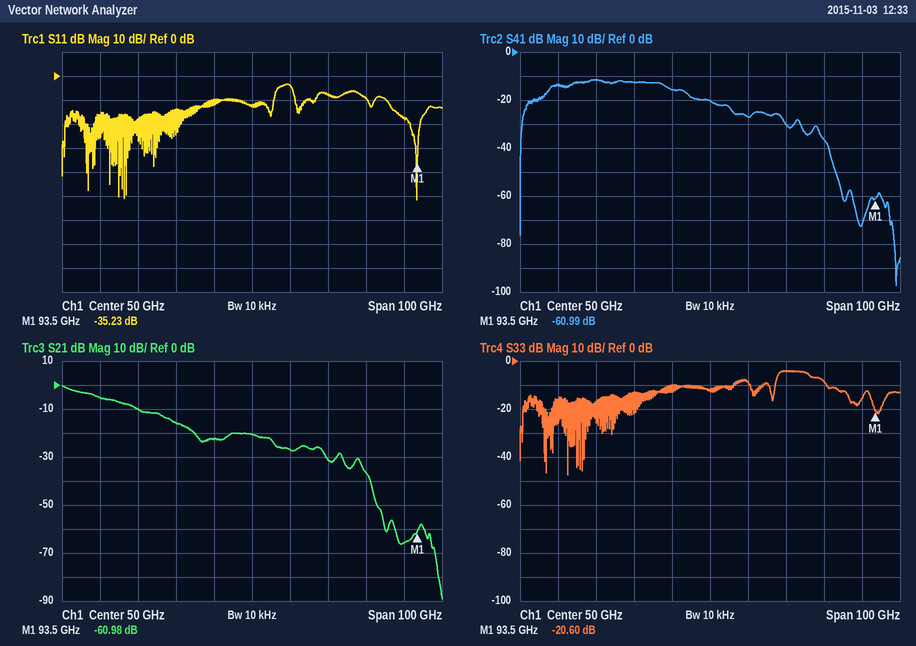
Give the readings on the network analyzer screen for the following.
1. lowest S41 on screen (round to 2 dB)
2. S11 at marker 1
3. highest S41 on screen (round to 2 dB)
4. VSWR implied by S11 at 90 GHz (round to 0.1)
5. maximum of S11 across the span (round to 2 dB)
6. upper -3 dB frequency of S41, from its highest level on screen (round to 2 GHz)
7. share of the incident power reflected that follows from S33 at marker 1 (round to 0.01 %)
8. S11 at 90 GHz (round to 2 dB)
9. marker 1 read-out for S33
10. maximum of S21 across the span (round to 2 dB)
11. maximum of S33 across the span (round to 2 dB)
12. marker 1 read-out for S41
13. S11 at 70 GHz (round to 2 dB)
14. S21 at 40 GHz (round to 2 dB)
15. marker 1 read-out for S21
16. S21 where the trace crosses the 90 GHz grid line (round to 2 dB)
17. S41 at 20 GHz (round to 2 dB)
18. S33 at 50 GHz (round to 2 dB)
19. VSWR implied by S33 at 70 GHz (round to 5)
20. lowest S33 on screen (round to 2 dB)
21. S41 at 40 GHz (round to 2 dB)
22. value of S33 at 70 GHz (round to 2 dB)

-98 dB
-35.23 dB
-12 dB
1.3
-4 dB
38 GHz
0.87 %
-18 dB
-20.60 dB
0 dB
-4 dB
-60.99 dB
-8 dB
-22 dB
-60.98 dB
-66 dB
-12 dB
-12 dB
5
-48 dB
-16 dB
-4 dB
